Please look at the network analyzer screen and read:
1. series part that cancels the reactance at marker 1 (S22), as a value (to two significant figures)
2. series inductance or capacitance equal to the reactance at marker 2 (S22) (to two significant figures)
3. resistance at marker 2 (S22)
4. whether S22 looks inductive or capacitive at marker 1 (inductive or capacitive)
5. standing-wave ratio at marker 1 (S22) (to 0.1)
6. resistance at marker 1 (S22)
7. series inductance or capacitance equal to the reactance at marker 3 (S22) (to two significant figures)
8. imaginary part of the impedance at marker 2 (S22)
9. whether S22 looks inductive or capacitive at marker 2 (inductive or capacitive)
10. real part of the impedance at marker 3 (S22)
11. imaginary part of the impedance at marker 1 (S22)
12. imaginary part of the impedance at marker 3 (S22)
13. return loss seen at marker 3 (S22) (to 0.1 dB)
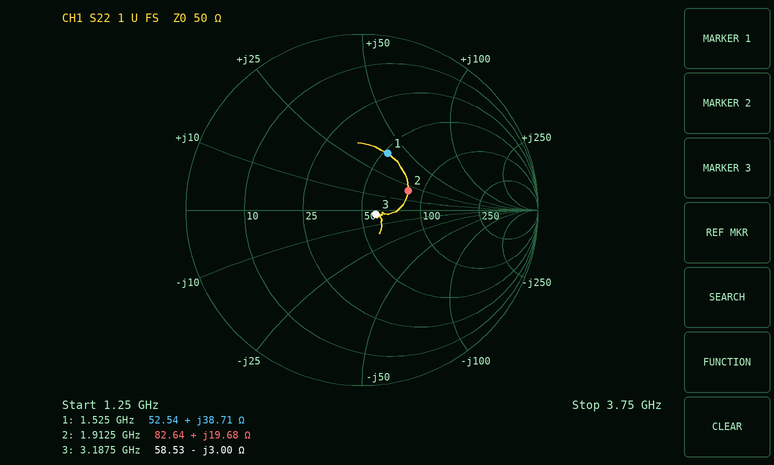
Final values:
2.7 pF
1.6 nH
82.64 Ω
inductive
2.1
52.54 Ω
17 pF
+19.68 Ω
inductive
58.53 Ω
+38.71 Ω
-3.00 Ω
21.6 dB
